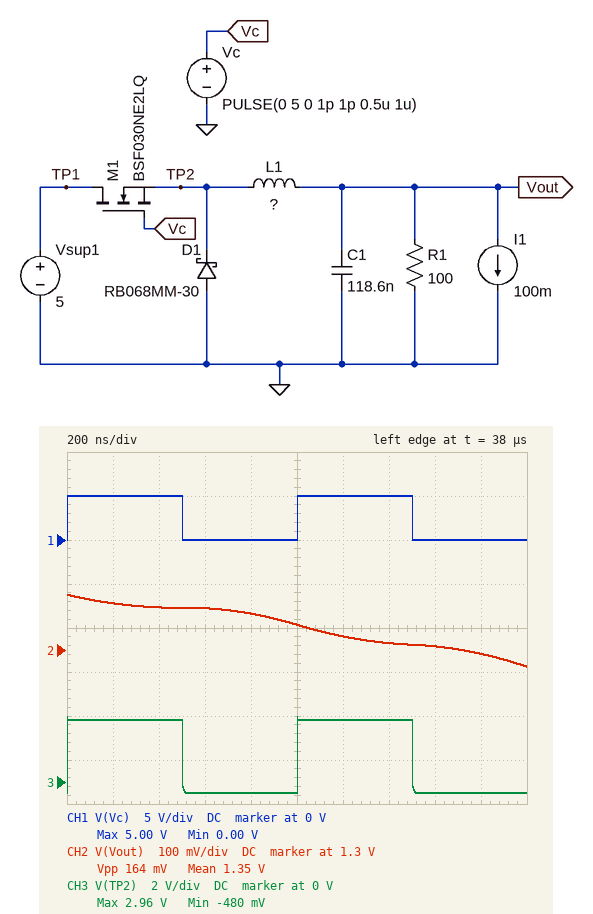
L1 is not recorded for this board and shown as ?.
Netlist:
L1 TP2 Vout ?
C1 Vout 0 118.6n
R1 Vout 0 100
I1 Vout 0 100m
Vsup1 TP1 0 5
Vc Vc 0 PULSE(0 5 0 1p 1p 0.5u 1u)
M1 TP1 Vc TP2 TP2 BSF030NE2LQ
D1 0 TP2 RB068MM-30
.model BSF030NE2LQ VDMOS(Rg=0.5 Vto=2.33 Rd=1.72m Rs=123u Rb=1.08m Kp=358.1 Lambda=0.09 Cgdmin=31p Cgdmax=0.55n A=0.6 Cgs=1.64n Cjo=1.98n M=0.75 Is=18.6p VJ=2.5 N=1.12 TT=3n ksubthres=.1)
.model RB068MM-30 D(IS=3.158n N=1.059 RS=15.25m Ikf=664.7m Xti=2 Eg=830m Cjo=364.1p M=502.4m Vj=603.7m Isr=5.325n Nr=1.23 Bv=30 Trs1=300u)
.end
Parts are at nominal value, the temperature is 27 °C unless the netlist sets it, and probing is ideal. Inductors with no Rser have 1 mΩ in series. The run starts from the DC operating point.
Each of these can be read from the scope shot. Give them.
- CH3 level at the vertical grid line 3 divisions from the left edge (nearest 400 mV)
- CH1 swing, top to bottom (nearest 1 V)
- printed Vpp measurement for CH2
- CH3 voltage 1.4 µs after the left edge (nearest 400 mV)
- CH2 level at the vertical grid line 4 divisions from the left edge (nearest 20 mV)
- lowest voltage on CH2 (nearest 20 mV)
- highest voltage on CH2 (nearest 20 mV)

-400 mV
5 V
164 mV
2.8 V
1.38 V
1.26 V
1.42 V
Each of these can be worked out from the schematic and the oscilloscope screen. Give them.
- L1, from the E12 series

47 µH
